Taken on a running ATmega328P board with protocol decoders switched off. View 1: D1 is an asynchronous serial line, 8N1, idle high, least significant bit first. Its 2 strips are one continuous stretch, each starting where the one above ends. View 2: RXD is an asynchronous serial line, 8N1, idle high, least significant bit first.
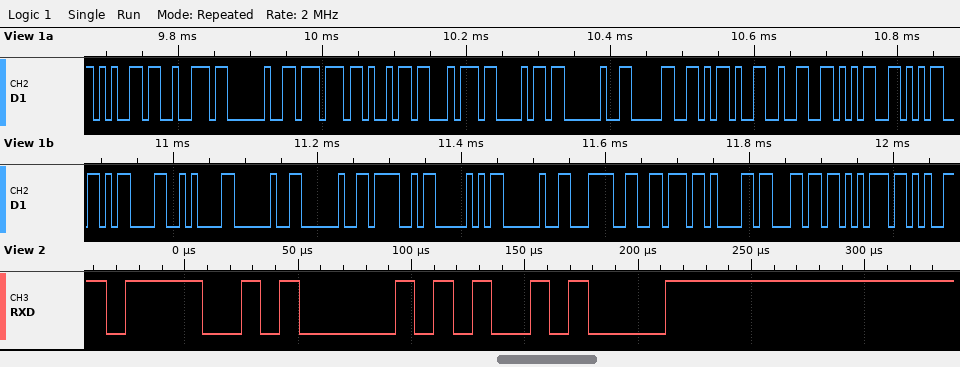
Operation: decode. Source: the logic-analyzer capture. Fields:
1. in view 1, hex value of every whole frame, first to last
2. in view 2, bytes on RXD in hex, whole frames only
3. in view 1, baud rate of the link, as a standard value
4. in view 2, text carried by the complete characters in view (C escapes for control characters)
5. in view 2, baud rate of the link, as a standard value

0x65 0x72 0x20 0x77 0x69 0x74 0x68 0x20 0x30 0x2D 0x32 0x35 0x35 0x0D 0x0A 0x20 0x20 0x4F 0x50 0x20 0x3C 0x76 0x61 0x6C 0x75
4F 50 0A
115200 baud
"OP\n"
115200 baud
